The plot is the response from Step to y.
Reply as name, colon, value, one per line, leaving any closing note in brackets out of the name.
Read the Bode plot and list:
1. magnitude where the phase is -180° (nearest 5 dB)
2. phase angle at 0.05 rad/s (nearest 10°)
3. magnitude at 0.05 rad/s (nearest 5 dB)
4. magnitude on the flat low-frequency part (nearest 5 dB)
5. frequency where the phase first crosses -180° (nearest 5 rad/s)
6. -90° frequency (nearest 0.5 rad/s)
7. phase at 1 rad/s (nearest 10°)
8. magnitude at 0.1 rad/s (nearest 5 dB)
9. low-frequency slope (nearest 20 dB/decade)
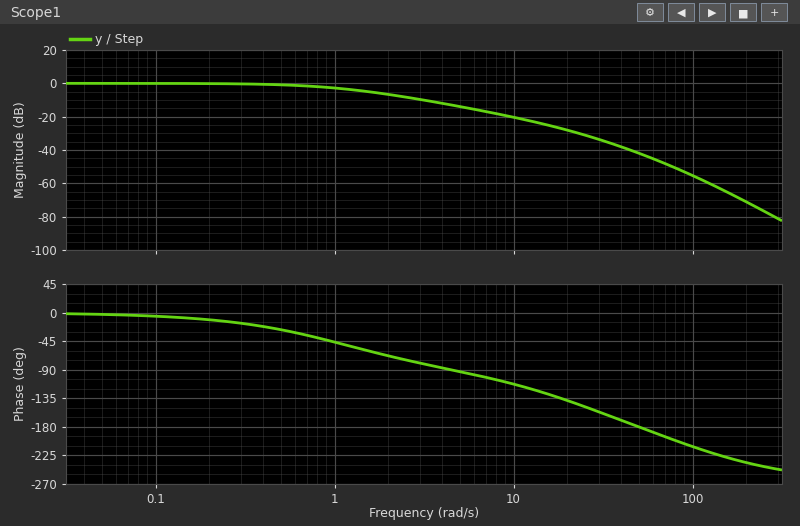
magnitude where the phase is -180°: -40 dB
phase angle at 0.05 rad/s: 0°
magnitude at 0.05 rad/s: 0 dB
magnitude on the flat low-frequency part: 0 dB
frequency where the phase first crosses -180°: 50 rad/s
-90° frequency: 4.5 rad/s
phase at 1 rad/s: -50°
magnitude at 0.1 rad/s: 0 dB
low-frequency slope: 0 dB/decade
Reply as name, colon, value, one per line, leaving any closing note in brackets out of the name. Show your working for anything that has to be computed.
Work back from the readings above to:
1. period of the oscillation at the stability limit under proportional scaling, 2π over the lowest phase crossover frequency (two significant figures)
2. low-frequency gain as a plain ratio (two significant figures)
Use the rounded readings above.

period of the oscillation at the stability limit under proportional scaling, 2π over the lowest phase crossover frequency: 2π / 50 = 0.13 s
low-frequency gain as a plain ratio: 10^(0 / 20) = 1.0
